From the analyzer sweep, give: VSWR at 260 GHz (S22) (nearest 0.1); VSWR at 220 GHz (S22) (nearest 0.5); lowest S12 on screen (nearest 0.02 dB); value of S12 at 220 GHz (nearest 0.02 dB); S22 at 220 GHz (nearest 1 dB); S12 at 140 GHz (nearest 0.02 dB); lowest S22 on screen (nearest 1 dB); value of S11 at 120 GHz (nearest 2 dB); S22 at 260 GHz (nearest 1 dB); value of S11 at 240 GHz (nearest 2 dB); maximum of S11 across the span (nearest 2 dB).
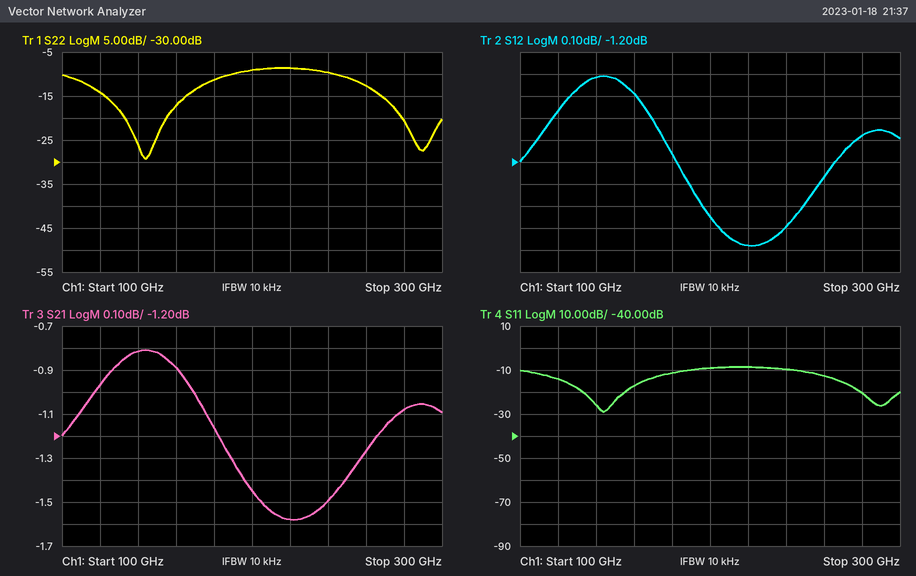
1.6
2.0
-1.58 dB
-1.58 dB
-9 dB
-0.82 dB
-29 dB
-14 dB
-13 dB
-10 dB
-8 dB
